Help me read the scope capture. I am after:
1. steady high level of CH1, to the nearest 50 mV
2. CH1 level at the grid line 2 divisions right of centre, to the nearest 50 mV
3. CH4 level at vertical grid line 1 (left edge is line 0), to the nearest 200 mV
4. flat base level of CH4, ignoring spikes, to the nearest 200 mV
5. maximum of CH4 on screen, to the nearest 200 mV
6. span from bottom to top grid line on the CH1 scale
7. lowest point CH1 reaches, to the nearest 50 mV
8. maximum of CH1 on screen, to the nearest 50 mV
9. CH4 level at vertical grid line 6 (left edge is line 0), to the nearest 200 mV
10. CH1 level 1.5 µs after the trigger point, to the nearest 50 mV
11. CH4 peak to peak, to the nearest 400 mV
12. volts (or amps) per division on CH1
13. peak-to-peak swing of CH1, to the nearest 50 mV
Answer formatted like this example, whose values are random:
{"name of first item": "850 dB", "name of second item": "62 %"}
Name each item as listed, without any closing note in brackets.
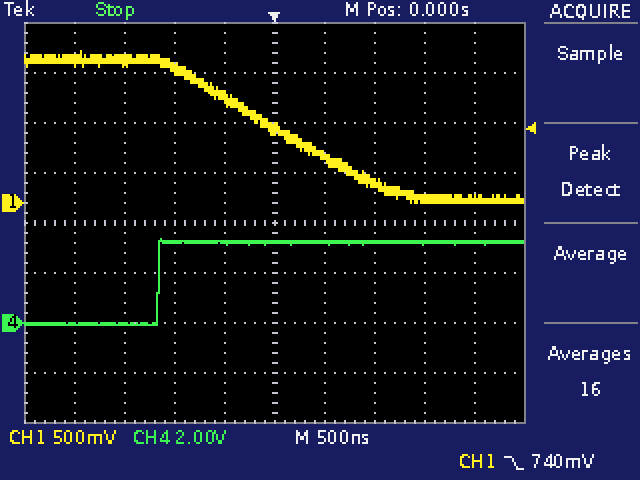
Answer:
{"steady high level of CH1, to the nearest 50 mV": "1.45 V", "CH1 level at the grid line 2 divisions right of centre, to the nearest 50 mV": "200 mV", "CH4 level at vertical grid line 1 (left edge is line 0), to the nearest 200 mV": "0.0 V", "flat base level of CH4, ignoring spikes, to the nearest 200 mV": "0.0 V", "maximum of CH4 on screen, to the nearest 200 mV": "3.4 V", "span from bottom to top grid line on the CH1 scale": "4 V", "lowest point CH1 reaches, to the nearest 50 mV": "0 mV", "maximum of CH1 on screen, to the nearest 50 mV": "1.50 V", "CH4 level at vertical grid line 6 (left edge is line 0), to the nearest 200 mV": "3.2 V", "CH1 level 1.5 µs after the trigger point, to the nearest 50 mV": "50 mV", "CH4 peak to peak, to the nearest 400 mV": "3.6 V", "volts (or amps) per division on CH1": "500 mV", "peak-to-peak swing of CH1, to the nearest 50 mV": "1.50 V"}
